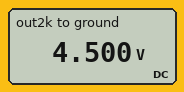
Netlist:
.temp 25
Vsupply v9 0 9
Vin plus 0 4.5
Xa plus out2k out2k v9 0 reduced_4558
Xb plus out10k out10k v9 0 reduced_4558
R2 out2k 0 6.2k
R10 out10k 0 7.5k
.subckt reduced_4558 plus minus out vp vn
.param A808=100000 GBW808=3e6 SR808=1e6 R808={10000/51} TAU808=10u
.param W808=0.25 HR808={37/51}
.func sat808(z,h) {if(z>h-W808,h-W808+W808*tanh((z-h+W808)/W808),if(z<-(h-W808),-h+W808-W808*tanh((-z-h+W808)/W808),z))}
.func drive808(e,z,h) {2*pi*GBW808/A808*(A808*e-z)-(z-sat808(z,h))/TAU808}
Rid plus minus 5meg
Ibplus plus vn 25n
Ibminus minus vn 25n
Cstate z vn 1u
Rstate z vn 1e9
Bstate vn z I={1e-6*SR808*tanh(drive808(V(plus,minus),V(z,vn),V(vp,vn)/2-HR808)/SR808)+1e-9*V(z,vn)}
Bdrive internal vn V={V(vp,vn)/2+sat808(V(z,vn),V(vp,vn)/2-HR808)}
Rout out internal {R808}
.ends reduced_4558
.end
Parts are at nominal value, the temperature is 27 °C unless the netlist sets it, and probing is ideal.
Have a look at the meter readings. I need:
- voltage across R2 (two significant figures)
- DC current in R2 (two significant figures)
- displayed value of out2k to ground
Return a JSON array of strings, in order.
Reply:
["4.5 V", "730 µA", "4.500 V"]
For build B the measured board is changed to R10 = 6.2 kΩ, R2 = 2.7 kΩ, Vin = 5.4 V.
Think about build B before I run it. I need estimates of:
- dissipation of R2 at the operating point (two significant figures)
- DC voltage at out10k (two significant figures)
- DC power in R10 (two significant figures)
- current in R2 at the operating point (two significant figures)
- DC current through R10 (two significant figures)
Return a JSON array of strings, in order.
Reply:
["11 mW", "5.4 V", "4.7 mW", "2.0 mA", "870 µA"]
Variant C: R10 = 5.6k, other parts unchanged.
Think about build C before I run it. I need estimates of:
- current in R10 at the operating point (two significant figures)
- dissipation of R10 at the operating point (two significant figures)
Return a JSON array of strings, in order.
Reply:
["800 µA", "3.6 mW"]
